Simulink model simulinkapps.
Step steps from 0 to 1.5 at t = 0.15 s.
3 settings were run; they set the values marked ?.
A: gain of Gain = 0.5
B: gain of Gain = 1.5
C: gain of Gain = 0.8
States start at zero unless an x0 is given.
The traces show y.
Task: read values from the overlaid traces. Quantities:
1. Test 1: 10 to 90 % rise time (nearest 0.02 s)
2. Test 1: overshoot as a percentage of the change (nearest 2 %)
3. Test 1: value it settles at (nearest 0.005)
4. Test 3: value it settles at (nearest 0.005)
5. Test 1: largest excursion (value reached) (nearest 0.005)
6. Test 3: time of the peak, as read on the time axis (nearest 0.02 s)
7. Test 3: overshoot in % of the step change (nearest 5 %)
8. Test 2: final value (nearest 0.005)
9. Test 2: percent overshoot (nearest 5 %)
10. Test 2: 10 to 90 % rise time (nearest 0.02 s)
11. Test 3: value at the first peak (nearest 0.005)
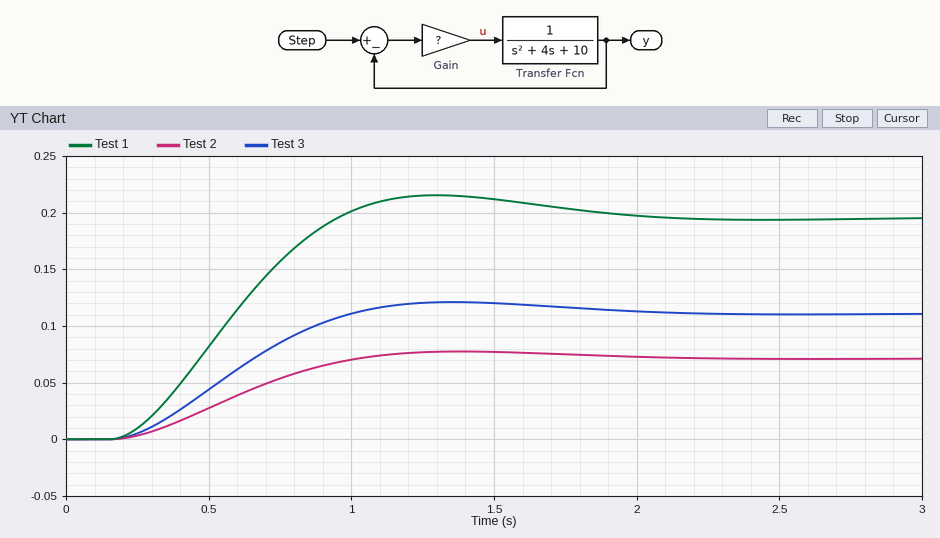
0.54 s
10 %
0.195
0.110
0.215
1.36 s
10 %
0.070
10 %
0.58 s
0.120
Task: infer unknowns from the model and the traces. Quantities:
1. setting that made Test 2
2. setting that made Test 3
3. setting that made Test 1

A
C
B
